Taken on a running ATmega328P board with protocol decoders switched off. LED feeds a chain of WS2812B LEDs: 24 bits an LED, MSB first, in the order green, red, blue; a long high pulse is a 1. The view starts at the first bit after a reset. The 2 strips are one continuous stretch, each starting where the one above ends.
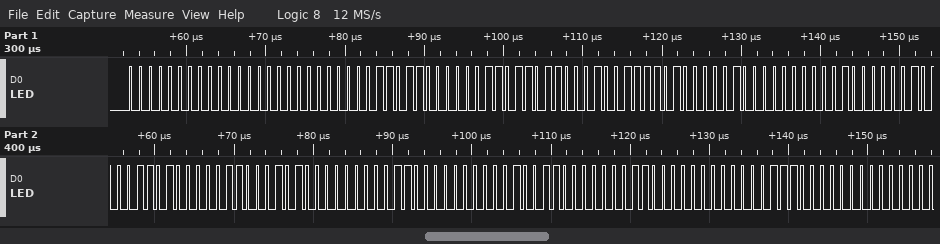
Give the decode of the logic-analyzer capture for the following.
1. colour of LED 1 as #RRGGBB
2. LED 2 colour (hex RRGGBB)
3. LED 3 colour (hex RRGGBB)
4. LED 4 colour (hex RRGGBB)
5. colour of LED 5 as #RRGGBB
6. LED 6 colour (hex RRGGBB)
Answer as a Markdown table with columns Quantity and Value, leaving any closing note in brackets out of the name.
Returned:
| Quantity | Value |
|---|---|
| colour of LED 1 as #RRGGBB | #000000 |
| LED 2 colour | #0D6CB1 |
| LED 3 colour | #043D00 |
| LED 4 colour | #0D8106 |
| colour of LED 5 as #RRGGBB | #032800 |
| LED 6 colour | #032600 |
